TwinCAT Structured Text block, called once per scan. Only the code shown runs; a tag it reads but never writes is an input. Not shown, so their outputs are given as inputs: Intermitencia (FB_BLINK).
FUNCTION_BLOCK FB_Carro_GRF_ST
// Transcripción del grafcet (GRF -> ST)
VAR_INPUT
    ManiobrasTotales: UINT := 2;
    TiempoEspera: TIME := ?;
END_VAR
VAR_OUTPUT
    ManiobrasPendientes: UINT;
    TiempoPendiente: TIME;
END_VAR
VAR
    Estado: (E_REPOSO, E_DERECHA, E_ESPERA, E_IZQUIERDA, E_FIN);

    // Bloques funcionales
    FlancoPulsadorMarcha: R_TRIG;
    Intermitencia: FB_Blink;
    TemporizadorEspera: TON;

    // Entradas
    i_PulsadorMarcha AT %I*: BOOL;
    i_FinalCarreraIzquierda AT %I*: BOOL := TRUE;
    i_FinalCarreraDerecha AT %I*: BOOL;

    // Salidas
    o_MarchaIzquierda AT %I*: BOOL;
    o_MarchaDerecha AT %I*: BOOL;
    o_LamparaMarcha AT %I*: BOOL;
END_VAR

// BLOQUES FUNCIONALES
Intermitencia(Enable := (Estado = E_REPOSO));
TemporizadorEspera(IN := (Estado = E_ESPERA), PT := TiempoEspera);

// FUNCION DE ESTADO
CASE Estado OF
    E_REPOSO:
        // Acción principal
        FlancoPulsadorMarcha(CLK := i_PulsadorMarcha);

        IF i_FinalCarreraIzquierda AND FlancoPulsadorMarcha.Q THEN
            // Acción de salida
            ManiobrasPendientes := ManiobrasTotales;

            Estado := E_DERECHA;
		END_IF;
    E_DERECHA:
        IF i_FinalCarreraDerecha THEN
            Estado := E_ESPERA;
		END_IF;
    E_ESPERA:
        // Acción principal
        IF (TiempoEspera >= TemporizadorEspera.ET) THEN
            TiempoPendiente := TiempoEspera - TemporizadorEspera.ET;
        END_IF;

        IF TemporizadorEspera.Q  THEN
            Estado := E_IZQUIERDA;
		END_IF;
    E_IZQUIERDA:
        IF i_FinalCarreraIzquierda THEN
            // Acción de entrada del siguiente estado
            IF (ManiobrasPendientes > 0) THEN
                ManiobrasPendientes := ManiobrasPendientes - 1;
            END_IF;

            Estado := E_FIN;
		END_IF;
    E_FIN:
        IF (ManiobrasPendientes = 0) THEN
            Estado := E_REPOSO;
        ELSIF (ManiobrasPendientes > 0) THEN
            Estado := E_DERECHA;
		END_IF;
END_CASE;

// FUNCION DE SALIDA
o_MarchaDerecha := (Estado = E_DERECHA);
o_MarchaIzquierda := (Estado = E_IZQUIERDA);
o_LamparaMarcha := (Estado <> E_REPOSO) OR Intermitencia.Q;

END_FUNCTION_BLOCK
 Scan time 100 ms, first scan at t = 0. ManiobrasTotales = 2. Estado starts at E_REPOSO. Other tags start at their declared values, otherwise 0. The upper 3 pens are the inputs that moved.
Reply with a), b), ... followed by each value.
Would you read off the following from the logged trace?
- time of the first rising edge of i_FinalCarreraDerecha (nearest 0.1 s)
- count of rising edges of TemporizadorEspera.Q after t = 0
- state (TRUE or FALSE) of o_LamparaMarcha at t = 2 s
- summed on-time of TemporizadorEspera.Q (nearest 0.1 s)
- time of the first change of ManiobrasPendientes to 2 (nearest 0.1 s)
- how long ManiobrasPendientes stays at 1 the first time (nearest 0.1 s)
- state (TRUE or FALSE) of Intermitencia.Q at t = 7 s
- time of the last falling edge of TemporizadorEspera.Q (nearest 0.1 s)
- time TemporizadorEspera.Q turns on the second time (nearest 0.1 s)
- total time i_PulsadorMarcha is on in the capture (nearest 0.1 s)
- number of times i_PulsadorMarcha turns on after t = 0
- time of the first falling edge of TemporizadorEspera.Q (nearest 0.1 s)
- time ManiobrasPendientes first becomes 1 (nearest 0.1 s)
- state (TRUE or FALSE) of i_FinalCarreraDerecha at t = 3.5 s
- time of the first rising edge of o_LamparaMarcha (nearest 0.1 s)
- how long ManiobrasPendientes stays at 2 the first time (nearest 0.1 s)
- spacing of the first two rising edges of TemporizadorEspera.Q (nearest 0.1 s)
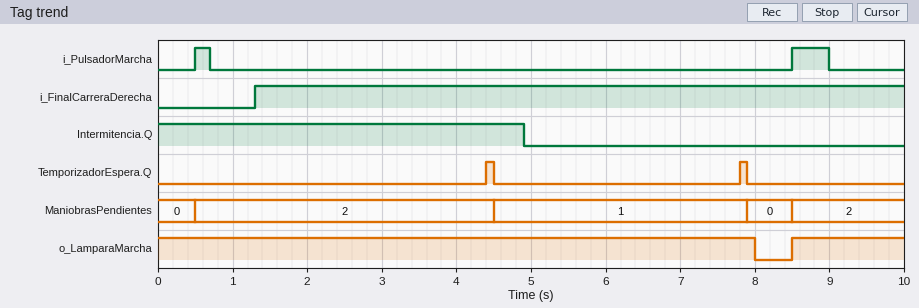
a) 1.3 s
b) 2
c) TRUE
d) 0.2 s
e) 0.5 s
f) 3.4 s
g) FALSE
h) 7.9 s
i) 7.8 s
j) 0.7 s
k) 2
l) 4.5 s
m) 4.5 s
n) TRUE
o) 8.5 s
p) 4.0 s
q) 3.4 s
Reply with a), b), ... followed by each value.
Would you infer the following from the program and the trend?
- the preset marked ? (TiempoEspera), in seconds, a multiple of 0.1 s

a) 3.0 s
